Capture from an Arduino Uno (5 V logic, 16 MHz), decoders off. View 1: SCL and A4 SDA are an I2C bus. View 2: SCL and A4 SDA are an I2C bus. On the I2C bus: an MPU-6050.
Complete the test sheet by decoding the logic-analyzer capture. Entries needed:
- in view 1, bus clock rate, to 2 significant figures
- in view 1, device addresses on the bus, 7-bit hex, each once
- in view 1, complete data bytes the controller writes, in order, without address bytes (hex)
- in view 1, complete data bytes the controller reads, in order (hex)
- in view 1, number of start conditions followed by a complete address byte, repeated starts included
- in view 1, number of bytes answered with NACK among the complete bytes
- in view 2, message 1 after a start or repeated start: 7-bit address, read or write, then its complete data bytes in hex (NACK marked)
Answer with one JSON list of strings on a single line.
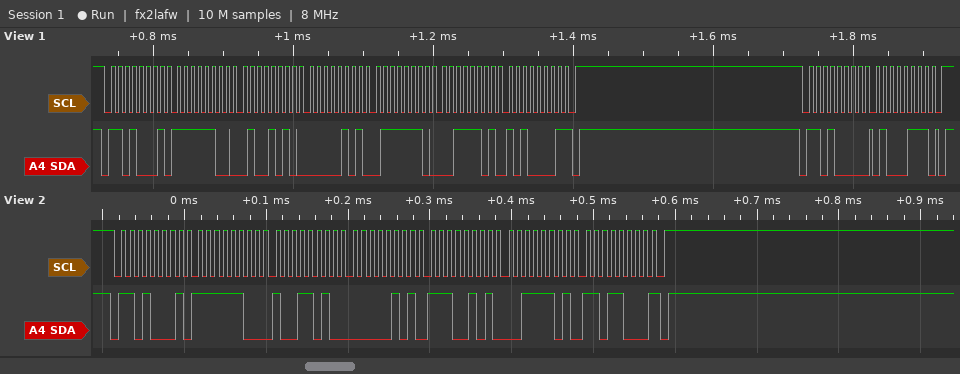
["100 kHz", "0x68", "47", "FC 4A 05 7E 3D A1", "2", "1", "0x68 read: FC 9A 05 E5 3D D8 NACK"]
